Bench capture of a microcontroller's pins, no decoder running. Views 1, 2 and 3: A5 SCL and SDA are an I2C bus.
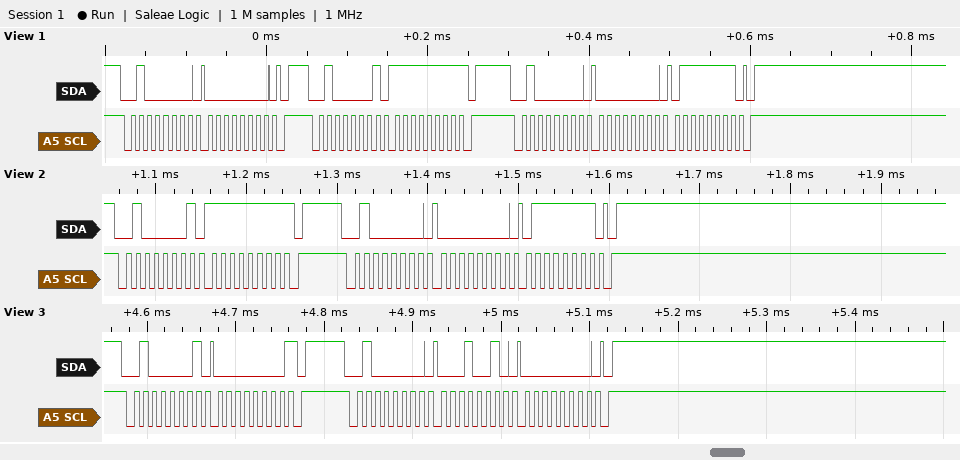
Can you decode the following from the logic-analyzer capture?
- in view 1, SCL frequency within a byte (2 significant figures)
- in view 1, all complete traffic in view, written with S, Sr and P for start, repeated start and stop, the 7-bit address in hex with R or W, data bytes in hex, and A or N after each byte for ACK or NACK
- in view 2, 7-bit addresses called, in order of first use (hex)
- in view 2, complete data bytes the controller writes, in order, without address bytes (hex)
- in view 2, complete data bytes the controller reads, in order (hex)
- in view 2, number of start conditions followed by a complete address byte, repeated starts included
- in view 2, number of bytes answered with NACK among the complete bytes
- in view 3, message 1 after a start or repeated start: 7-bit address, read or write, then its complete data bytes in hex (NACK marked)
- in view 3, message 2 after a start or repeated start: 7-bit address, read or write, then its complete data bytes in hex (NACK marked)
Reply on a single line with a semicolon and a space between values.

100 kHz; S 20W A 00 A P S 20R A FF N P S 20W A 00 A 7F A P; 0x20; 00 7F; FF; 2; 1; 0x20 read: 00 NACK; 0x20 write: 12 00
